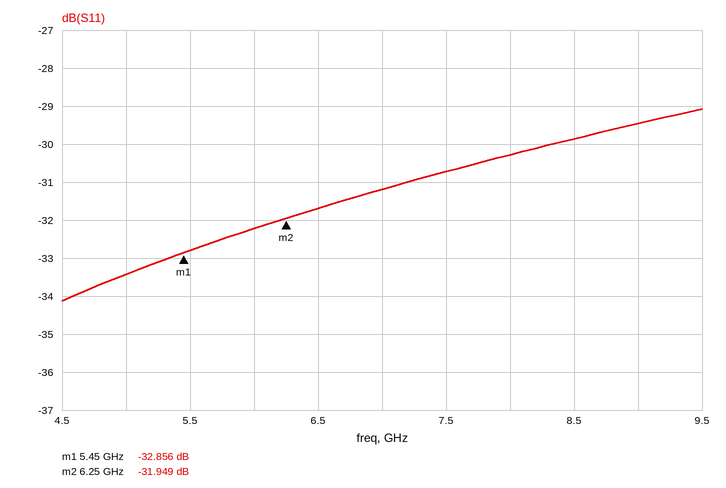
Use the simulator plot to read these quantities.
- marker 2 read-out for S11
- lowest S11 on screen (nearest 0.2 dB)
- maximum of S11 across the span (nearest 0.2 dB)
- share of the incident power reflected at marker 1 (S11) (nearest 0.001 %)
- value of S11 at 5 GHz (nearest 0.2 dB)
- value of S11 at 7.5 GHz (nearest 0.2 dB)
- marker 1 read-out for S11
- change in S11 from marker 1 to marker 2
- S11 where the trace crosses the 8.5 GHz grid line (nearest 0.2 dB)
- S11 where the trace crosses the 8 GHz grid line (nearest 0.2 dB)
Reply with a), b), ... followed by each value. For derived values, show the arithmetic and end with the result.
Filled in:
a) -31.949 dB
b) -34.2 dB
c) -29.0 dB
d) 10^(-32.856/10) ≈ 0.052 %
e) -33.4 dB
f) -30.8 dB
g) -32.856 dB
h) -31.949 − (-32.856) = 0.907 dB
i) -29.8 dB
j) -30.2 dB
